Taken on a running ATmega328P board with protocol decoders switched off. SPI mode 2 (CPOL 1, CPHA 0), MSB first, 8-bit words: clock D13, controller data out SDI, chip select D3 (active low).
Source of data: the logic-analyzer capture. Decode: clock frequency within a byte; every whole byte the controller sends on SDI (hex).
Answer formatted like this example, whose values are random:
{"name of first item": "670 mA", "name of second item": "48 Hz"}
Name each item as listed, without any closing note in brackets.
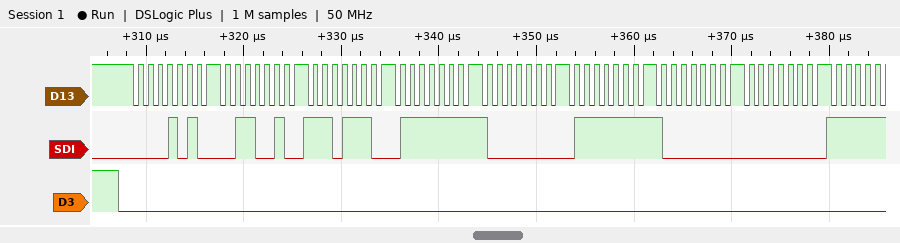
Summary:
{"clock frequency within a byte": "1 MHz", "every whole byte the controller sends on SDI": "0A 32 EE 7F 80 7F 80 00"}
